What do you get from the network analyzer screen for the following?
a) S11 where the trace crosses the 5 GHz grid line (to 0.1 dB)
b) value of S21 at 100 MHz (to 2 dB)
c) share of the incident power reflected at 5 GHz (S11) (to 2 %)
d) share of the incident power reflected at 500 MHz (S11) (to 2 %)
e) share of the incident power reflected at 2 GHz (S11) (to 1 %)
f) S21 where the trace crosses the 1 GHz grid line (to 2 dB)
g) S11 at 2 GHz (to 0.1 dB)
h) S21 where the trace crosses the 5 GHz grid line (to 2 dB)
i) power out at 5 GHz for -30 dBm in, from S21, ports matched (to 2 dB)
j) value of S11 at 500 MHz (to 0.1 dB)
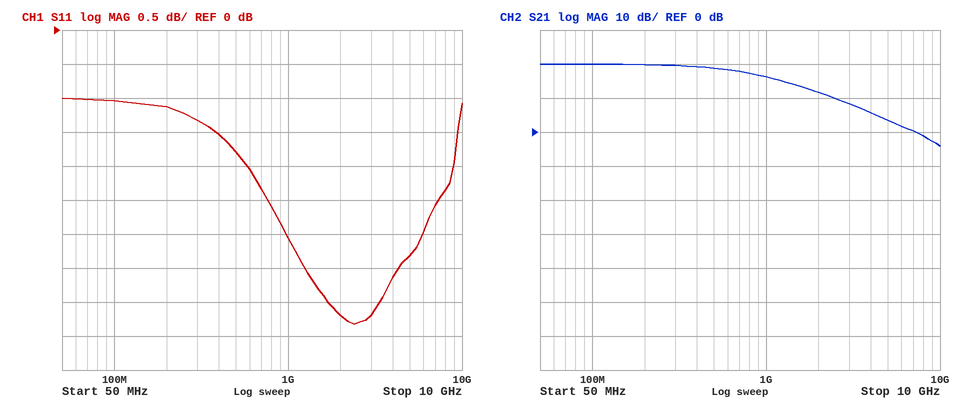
-3.3 dB
20 dB
46 %
66 %
38 %
16 dB
-4.2 dB
4 dB
-26 dBm
-1.8 dB
